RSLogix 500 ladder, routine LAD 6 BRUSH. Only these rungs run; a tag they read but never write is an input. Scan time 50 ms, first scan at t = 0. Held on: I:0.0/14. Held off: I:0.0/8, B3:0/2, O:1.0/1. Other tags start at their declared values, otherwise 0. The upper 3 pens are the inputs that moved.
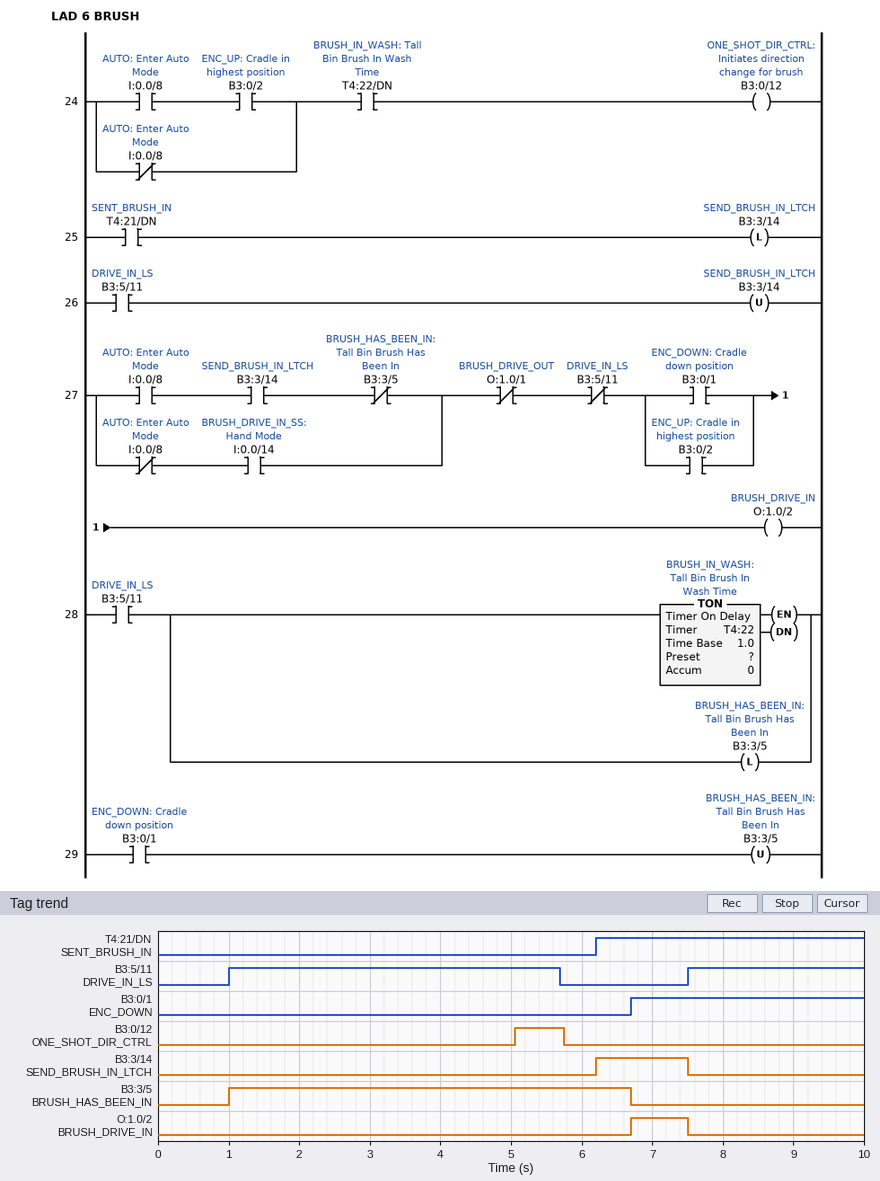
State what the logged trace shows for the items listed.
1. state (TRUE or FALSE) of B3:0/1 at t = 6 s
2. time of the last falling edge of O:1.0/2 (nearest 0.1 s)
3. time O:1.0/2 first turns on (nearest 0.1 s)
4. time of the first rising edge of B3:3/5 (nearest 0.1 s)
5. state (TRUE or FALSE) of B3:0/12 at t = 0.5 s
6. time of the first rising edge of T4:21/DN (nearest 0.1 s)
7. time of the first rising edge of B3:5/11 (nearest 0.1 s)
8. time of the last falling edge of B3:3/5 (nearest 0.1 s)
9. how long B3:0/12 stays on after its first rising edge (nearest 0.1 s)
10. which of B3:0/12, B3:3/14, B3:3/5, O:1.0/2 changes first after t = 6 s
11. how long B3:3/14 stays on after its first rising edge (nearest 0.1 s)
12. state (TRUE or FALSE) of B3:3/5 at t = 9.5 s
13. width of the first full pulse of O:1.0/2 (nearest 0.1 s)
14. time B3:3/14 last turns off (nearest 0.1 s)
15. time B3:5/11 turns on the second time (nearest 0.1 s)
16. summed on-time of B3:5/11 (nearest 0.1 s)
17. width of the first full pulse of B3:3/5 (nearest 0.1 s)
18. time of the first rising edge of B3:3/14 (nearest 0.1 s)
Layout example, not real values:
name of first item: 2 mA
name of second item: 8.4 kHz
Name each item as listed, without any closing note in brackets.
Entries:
state (TRUE or FALSE) of B3:0/1 at t = 6 s: FALSE
time of the last falling edge of O:1.0/2: 7.5 s
time O:1.0/2 first turns on: 6.7 s
time of the first rising edge of B3:3/5: 1.0 s
state (TRUE or FALSE) of B3:0/12 at t = 0.5 s: FALSE
time of the first rising edge of T4:21/DN: 6.2 s
time of the first rising edge of B3:5/11: 1.0 s
time of the last falling edge of B3:3/5: 6.7 s
how long B3:0/12 stays on after its first rising edge: 0.7 s
which of B3:0/12, B3:3/14, B3:3/5, O:1.0/2 changes first after t = 6 s: B3:3/14
how long B3:3/14 stays on after its first rising edge: 1.3 s
state (TRUE or FALSE) of B3:3/5 at t = 9.5 s: FALSE
width of the first full pulse of O:1.0/2: 0.8 s
time B3:3/14 last turns off: 7.5 s
time B3:5/11 turns on the second time: 7.5 s
summed on-time of B3:5/11: 7.2 s
width of the first full pulse of B3:3/5: 5.7 s
time of the first rising edge of B3:3/14: 6.2 s
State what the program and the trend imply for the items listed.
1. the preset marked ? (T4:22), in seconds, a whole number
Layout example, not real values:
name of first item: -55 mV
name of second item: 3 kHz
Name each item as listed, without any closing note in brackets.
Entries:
the preset marked ? (T4:22), in seconds, a whole number: 4 s
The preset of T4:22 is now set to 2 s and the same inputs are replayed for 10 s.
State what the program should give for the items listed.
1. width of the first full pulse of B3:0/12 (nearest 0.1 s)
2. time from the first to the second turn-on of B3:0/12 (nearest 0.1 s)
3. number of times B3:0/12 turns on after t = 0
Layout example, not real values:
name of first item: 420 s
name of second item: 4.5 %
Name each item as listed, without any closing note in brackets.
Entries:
width of the first full pulse of B3:0/12: 2.7 s
time from the first to the second turn-on of B3:0/12: 6.5 s
number of times B3:0/12 turns on after t = 0: 2
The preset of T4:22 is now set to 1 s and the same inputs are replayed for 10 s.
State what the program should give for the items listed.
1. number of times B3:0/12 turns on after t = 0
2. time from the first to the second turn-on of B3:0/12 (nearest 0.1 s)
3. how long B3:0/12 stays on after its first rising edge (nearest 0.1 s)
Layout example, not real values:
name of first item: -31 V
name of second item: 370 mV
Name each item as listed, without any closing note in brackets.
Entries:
number of times B3:0/12 turns on after t = 0: 2
time from the first to the second turn-on of B3:0/12: 6.5 s
how long B3:0/12 stays on after its first rising edge: 3.7 s
